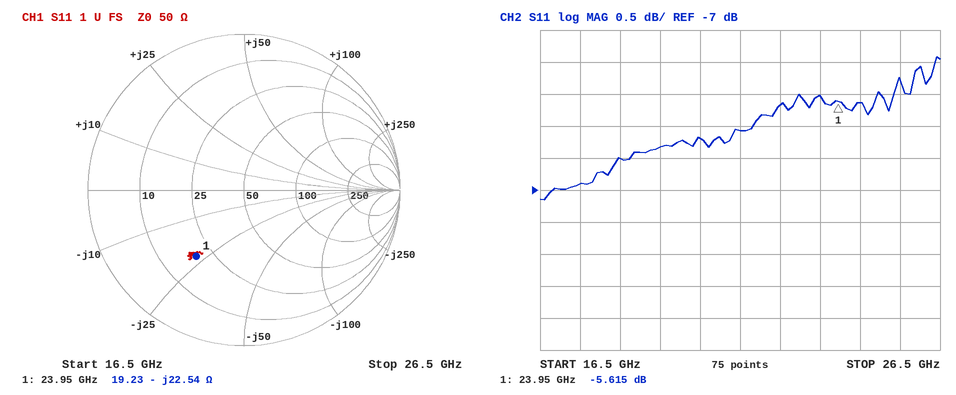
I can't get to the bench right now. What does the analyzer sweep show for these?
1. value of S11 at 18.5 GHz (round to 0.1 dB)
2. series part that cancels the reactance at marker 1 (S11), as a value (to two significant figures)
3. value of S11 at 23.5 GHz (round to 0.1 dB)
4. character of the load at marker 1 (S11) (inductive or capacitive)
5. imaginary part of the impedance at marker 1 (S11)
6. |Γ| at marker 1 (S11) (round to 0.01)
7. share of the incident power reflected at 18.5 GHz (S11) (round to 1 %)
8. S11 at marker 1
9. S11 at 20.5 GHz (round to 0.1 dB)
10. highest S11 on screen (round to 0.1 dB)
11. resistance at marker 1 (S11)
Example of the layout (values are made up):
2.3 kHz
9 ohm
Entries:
-6.5 dB
150 pH
-5.5 dB
capacitive
-22.54 Ω
0.52
22 %
-5.615 dB
-6.2 dB
-4.9 dB
19.23 Ω
